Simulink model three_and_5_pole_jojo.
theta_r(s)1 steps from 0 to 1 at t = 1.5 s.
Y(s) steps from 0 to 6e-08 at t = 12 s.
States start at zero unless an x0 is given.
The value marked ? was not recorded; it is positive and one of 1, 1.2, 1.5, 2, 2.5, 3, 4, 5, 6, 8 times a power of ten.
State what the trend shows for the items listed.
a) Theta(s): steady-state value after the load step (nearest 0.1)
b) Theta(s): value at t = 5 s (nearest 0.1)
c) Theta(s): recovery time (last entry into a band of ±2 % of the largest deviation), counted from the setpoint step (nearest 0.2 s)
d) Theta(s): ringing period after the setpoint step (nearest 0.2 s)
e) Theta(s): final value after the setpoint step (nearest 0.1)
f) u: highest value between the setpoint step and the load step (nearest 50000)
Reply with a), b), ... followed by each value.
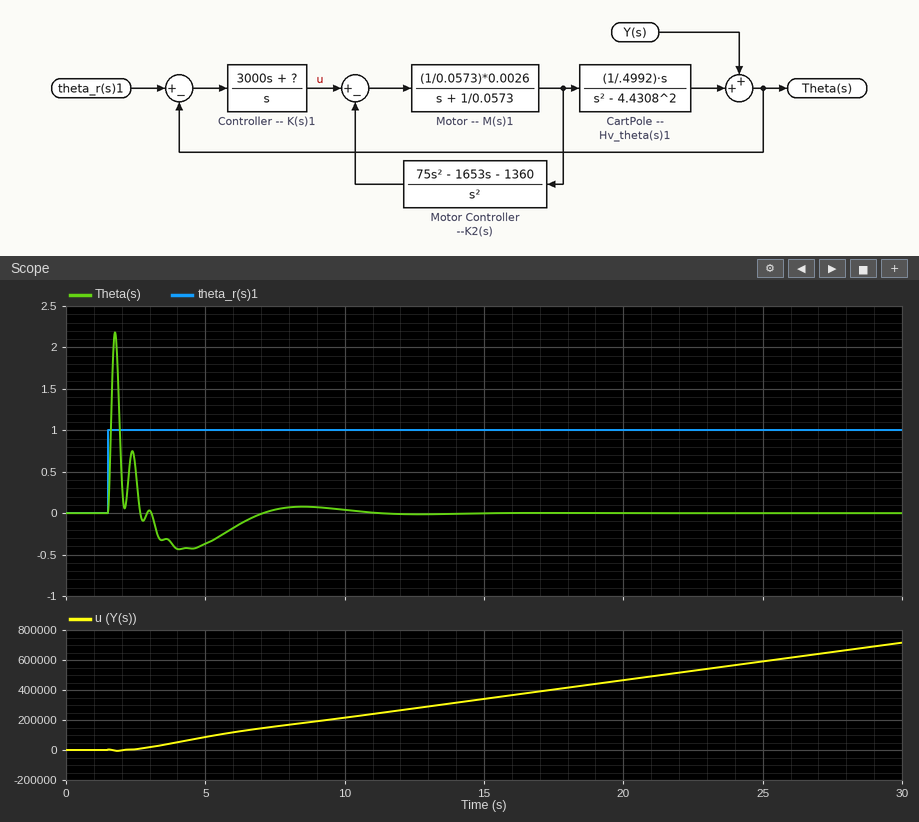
a) 0.0
b) -0.4
c) 8.4 s
d) 0.6 s
e) 0.0
f) 250000
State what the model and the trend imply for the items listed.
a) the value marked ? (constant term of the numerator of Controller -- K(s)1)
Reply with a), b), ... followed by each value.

a) 25000
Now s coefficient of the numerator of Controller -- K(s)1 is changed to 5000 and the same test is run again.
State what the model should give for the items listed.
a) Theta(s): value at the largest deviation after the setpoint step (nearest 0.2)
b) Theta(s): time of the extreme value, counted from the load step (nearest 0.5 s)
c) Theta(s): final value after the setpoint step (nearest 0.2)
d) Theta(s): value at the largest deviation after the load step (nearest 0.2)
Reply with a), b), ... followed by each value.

a) 1.8
b) 4.0 s
c) 0.0
d) 0.0
